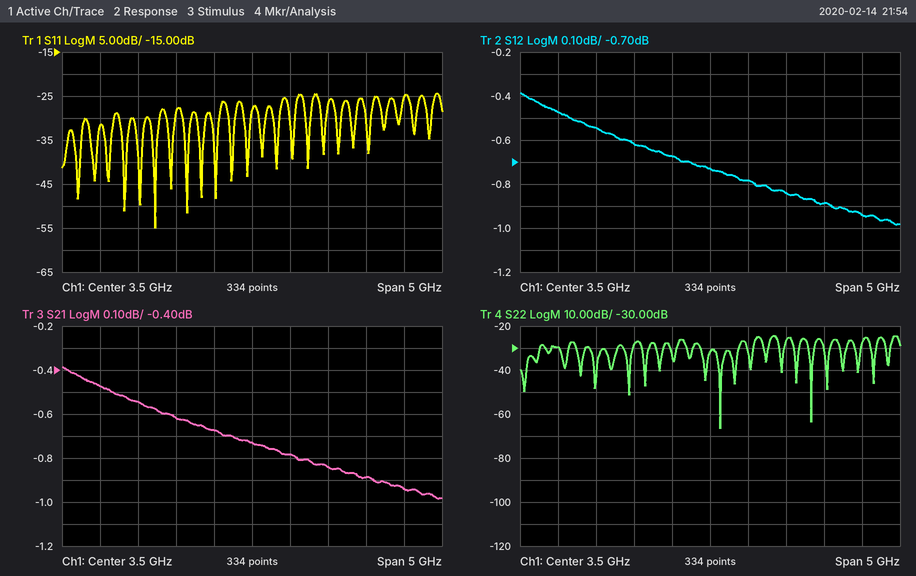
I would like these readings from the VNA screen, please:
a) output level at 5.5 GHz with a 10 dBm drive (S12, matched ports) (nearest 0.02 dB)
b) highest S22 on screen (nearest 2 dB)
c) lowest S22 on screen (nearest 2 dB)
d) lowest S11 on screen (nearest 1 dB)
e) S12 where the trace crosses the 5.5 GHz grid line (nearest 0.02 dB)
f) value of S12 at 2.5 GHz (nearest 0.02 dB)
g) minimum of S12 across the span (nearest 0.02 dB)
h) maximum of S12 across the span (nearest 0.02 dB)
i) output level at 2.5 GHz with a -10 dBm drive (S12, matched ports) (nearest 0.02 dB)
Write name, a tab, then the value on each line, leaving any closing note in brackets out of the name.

output level at 5.5 GHz with a 10 dBm drive (S12, matched ports)	9.06 dBm
highest S22 on screen	-24 dB
lowest S22 on screen	-66 dB
lowest S11 on screen	-55 dB
S12 where the trace crosses the 5.5 GHz grid line	-0.94 dB
value of S12 at 2.5 GHz	-0.62 dB
minimum of S12 across the span	-0.98 dB
maximum of S12 across the span	-0.38 dB
output level at 2.5 GHz with a -10 dBm drive (S12, matched ports)	-10.62 dBm
